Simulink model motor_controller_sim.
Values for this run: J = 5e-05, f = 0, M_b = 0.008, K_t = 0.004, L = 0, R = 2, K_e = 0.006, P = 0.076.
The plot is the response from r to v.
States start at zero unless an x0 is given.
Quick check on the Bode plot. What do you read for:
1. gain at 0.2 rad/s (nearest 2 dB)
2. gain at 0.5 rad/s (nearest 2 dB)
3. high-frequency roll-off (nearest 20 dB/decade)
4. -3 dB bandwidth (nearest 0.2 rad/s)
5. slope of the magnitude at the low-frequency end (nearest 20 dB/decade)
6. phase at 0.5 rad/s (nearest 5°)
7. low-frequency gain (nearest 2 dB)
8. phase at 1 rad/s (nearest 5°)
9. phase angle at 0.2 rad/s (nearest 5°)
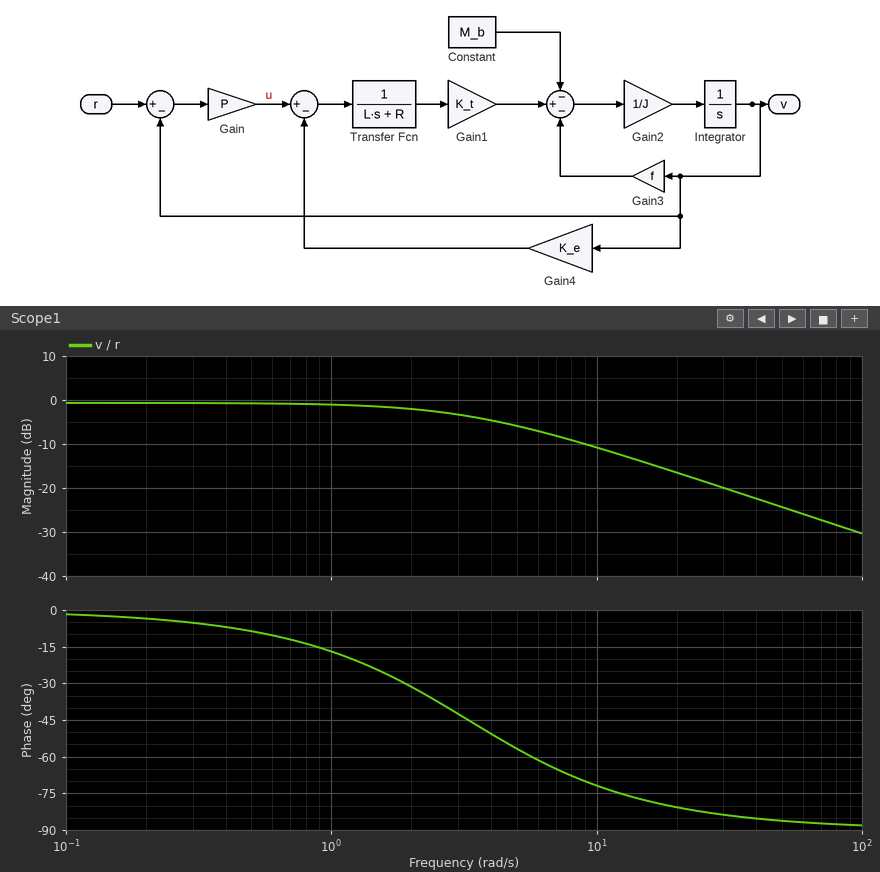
0 dB
0 dB
-20 dB/decade
3.2 rad/s
0 dB/decade
-10°
0 dB
-15°
-5°
